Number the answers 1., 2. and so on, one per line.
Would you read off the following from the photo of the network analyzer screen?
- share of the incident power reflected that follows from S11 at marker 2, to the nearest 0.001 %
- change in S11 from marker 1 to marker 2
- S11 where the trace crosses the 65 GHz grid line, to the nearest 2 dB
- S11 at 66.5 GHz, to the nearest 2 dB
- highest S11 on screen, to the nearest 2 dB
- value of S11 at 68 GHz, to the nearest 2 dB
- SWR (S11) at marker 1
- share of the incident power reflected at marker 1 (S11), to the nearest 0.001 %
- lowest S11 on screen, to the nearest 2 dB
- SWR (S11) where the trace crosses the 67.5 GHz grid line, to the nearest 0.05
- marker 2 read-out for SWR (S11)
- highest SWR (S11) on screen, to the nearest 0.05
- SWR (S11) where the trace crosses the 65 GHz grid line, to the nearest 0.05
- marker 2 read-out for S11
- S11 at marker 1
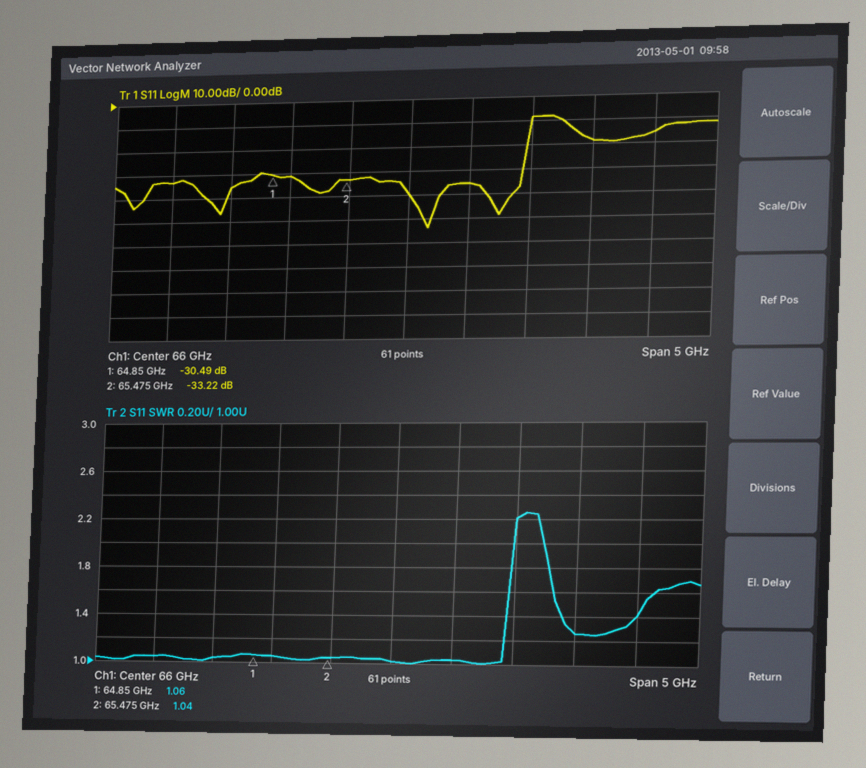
1. 0.048 %
2. -2.73 dB
3. -32 dB
4. -36 dB
5. -8 dB
6. -16 dB
7. 1.06
8. 0.089 %
9. -54 dB
10. 1.25
11. 1.04
12. 2.25
13. 1.05
14. -33.22 dB
15. -30.49 dB
